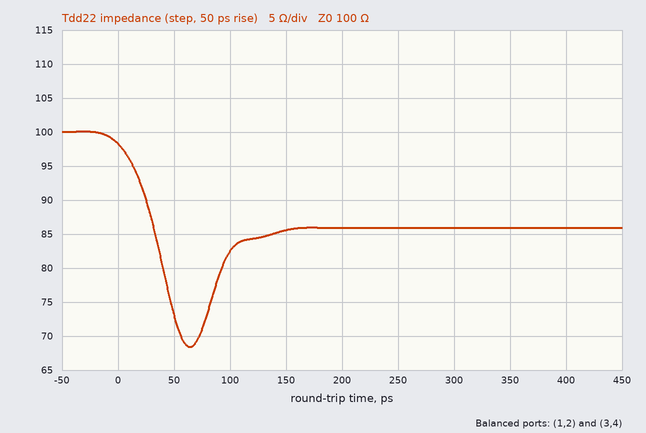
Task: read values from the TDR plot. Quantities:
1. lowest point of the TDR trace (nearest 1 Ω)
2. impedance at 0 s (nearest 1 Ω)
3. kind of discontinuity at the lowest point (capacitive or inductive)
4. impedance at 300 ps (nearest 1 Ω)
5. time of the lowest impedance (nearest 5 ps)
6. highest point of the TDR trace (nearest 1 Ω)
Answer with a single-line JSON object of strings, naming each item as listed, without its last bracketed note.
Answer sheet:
{"lowest point of the TDR trace": "68 Ω", "impedance at 0 s": "98 Ω", "kind of discontinuity at the lowest point": "capacitive", "impedance at 300 ps": "86 Ω", "time of the lowest impedance": "65 ps", "highest point of the TDR trace": "100 Ω"}
